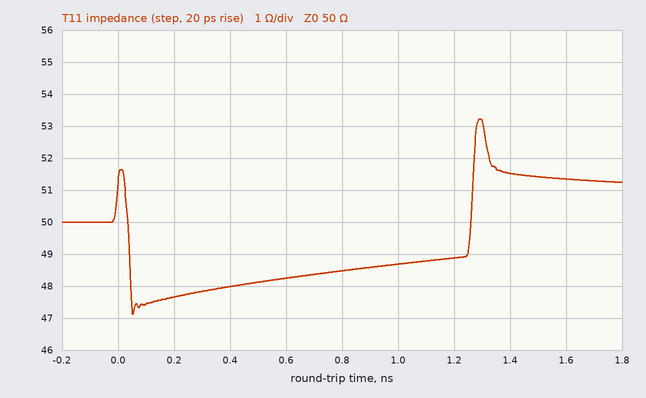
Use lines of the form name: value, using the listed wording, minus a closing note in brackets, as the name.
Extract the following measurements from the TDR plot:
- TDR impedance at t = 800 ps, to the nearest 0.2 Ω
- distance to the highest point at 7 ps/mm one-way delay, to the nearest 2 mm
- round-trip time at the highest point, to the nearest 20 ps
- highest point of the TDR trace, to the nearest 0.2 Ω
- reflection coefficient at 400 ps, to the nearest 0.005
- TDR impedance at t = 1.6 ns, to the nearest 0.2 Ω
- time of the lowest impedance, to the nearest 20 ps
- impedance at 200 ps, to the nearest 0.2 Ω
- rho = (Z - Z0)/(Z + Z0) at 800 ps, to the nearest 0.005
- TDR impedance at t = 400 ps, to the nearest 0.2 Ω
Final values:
TDR impedance at t = 800 ps, to the nearest 0.2 Ω: 48.4 Ω
distance to the highest point at 7 ps/mm one-way delay, to the nearest 2 mm: 92 mm
round-trip time at the highest point, to the nearest 20 ps: 1.30 ns
highest point of the TDR trace, to the nearest 0.2 Ω: 53.2 Ω
reflection coefficient at 400 ps, to the nearest 0.005: -0.020
TDR impedance at t = 1.6 ns, to the nearest 0.2 Ω: 51.4 Ω
time of the lowest impedance, to the nearest 20 ps: 60 ps
impedance at 200 ps, to the nearest 0.2 Ω: 47.6 Ω
rho = (Z - Z0)/(Z + Z0) at 800 ps, to the nearest 0.005: -0.015
TDR impedance at t = 400 ps, to the nearest 0.2 Ω: 48.0 Ω
